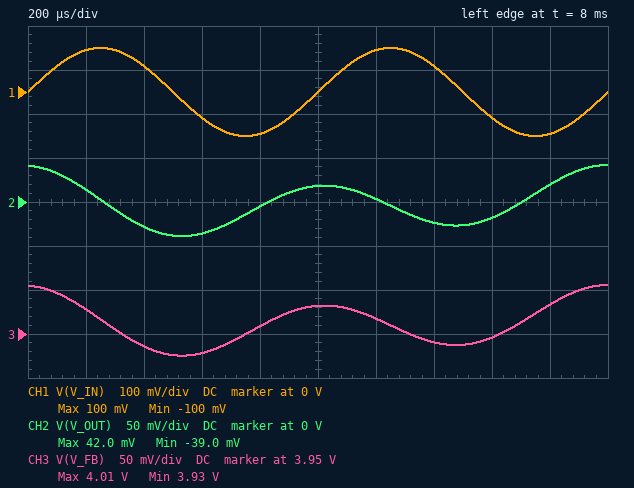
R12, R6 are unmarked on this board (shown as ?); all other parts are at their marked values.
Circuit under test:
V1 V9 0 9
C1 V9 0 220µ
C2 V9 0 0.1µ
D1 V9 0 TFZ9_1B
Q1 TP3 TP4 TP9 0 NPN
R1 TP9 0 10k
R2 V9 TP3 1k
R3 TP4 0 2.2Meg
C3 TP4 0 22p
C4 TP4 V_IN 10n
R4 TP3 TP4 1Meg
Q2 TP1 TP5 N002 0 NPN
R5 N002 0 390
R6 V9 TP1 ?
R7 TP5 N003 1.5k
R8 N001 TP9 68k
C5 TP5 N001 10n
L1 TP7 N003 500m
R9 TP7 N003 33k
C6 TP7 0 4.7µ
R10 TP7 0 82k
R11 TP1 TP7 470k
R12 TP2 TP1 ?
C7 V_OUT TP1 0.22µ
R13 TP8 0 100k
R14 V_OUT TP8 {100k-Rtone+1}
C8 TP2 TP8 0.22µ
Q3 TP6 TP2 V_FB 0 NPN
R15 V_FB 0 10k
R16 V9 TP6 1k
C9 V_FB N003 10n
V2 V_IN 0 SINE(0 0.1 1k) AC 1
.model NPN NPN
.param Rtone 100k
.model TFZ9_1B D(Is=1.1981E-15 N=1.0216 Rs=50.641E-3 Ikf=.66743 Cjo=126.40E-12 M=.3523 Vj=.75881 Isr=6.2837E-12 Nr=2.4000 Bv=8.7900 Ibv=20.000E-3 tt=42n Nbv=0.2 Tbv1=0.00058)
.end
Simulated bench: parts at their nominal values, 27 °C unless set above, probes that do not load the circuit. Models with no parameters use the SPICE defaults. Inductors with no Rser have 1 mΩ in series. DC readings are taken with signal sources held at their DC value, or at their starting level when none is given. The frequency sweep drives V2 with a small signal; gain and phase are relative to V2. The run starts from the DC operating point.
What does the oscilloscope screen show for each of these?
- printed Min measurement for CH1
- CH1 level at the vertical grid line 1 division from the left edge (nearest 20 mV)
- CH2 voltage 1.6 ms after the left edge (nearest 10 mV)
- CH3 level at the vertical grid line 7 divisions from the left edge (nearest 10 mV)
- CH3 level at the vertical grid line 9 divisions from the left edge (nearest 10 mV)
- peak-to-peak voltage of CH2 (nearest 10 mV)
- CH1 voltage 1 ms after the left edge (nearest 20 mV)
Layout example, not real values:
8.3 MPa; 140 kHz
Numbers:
-100 mV; 100 mV; -20 mV; 3.94 V; 3.98 V; 80 mV; 0 V
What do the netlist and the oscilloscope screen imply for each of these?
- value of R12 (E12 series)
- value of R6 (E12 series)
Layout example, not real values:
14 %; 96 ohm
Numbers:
330 kΩ; 18 kΩ
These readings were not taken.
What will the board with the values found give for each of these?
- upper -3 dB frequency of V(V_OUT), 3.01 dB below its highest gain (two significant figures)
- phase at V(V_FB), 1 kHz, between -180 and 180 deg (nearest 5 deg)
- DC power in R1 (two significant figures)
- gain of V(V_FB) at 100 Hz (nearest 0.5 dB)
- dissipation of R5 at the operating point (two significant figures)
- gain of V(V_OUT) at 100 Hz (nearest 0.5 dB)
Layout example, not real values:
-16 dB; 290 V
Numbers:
470 Hz; 90 deg; 970 µW; -14.0 dB; 9.1 µW; -14.0 dB
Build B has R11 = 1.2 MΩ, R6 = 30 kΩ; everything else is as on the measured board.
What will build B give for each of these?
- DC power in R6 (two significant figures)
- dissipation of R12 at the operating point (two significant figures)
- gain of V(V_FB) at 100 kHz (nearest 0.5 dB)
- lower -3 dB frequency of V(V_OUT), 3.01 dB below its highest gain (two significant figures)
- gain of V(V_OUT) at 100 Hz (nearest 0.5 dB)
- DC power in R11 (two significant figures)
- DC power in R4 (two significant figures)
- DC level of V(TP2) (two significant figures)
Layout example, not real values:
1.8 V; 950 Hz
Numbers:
4.9 µW; 11 µW; -66.0 dB; 1.8 kHz; -58.5 dB; 54 µW; 23 µW; 6.7 V
